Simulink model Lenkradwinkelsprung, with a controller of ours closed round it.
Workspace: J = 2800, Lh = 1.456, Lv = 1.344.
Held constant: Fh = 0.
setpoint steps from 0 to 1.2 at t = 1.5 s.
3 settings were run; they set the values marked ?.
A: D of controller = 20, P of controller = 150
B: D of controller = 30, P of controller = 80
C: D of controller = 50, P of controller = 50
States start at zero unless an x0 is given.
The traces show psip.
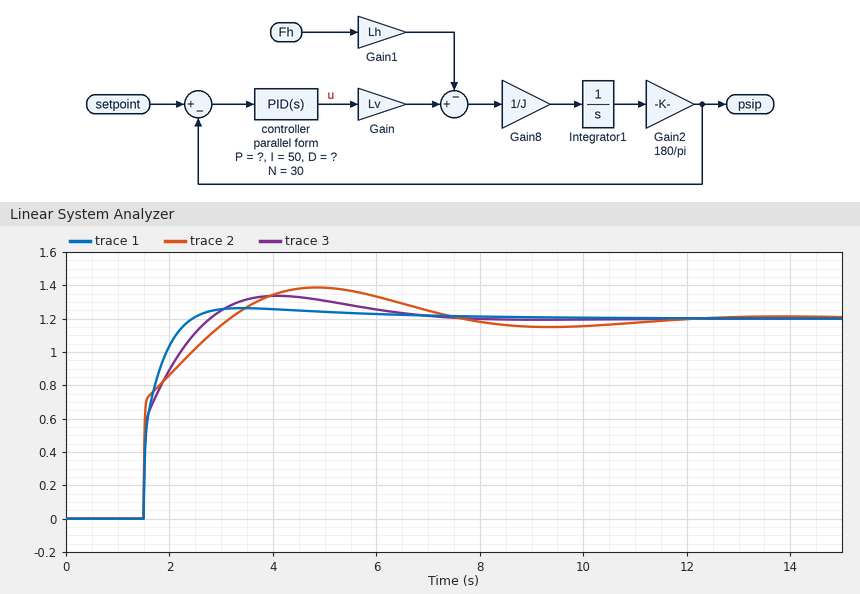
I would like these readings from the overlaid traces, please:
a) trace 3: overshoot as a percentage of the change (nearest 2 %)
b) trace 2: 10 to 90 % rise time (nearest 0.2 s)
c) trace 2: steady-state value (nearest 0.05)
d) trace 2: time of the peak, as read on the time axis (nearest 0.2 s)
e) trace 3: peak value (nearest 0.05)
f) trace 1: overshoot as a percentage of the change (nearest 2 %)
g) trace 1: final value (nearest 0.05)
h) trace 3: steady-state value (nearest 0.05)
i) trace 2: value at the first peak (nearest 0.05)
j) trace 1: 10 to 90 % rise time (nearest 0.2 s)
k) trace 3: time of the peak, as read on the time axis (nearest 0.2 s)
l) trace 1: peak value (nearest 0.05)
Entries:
12 %
1.2 s
1.20
4.8 s
1.35
6 %
1.20
1.20
1.40
0.6 s
4.0 s
1.25
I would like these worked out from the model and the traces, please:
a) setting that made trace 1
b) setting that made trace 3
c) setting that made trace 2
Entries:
A
B
C
